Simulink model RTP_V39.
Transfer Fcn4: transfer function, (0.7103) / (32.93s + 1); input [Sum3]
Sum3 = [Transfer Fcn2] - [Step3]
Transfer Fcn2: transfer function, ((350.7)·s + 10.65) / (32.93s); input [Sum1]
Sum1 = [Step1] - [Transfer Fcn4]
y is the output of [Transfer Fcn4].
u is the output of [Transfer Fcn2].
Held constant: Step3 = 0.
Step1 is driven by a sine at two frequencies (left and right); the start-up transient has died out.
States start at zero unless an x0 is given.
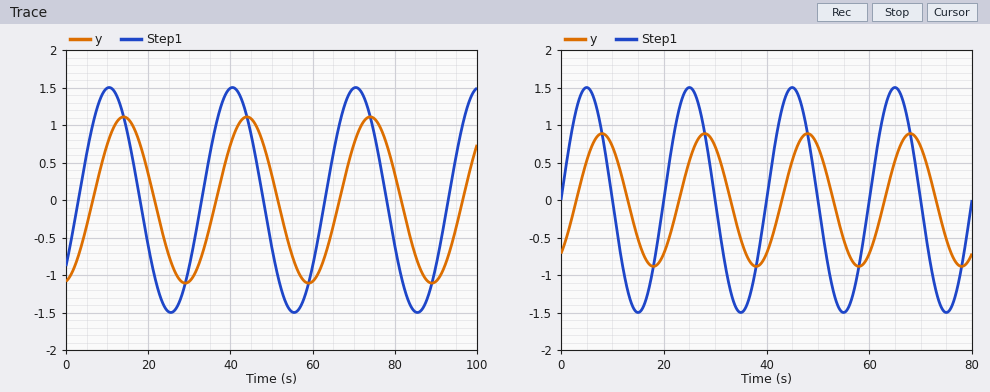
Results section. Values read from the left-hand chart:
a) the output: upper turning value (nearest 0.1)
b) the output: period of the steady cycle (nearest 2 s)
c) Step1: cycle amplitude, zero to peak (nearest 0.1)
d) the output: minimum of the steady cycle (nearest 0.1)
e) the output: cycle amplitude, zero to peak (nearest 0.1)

1.1
30 s
1.5
-1.1
1.1
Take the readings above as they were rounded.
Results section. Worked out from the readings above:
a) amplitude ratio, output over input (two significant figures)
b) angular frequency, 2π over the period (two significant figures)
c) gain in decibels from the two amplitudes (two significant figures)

0.73
0.21 rad/s
-2.7 dB
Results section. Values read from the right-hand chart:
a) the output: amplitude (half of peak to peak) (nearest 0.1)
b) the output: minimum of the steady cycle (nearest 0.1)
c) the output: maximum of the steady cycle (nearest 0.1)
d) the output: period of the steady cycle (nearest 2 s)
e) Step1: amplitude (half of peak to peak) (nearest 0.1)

0.9
-0.9
0.9
20 s
1.5
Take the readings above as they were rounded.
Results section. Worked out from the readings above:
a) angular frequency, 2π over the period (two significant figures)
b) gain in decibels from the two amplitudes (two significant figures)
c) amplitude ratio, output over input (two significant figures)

0.31 rad/s
-4.4 dB
0.60
